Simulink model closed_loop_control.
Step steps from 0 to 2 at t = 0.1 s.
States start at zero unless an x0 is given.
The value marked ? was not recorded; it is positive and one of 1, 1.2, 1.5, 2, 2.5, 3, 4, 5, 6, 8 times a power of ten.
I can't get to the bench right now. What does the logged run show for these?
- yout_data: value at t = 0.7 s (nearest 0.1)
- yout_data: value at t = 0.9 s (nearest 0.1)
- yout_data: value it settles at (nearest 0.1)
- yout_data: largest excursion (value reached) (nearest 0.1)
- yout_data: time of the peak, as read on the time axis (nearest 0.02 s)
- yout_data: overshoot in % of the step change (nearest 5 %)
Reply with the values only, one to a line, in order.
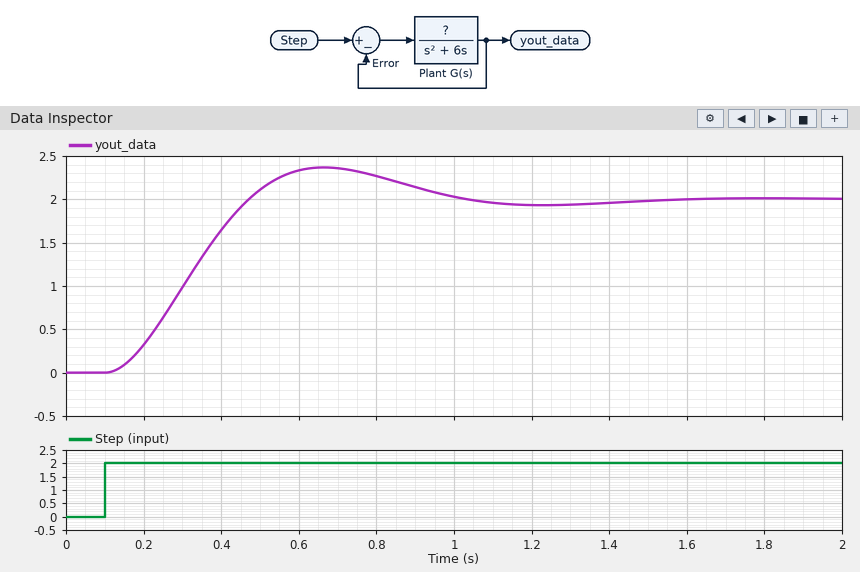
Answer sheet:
2.4
2.1
2.0
2.4
0.66 s
20 %
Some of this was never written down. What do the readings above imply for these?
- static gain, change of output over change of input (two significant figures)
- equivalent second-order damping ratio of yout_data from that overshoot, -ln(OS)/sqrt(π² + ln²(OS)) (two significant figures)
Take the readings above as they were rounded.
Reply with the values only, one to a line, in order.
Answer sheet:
1.0
0.46
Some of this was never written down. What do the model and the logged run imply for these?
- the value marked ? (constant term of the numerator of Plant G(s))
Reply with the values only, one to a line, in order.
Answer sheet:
40
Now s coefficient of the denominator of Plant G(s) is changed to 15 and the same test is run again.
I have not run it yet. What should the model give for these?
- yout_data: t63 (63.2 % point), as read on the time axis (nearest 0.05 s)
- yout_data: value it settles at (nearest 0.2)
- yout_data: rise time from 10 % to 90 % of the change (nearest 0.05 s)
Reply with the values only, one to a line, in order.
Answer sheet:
0.50 s
2.0
0.70 s
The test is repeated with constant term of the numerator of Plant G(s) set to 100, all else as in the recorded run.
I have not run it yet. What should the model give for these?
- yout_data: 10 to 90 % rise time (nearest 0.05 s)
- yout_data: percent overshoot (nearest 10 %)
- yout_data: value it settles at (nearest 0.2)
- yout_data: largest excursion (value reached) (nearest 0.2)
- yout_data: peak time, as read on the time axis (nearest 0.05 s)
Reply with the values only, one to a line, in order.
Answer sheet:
0.15 s
40 %
2.0
2.8
0.45 s
